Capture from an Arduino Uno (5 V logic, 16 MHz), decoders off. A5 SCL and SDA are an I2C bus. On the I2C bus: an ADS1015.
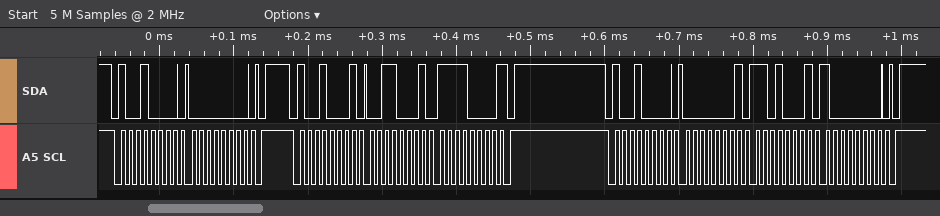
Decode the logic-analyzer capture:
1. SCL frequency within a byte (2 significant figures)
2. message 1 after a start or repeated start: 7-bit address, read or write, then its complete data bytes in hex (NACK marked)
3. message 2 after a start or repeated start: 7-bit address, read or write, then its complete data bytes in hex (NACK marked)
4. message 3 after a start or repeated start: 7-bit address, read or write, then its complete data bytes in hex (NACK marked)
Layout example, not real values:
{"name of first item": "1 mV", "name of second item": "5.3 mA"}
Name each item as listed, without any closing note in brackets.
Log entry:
{"SCL frequency within a byte": "100 kHz", "message 1 after a start or repeated start: 7-bit address, read or write, then its complete data bytes in hex": "0x48 write: 00", "message 2 after a start or repeated start: 7-bit address, read or write, then its complete data bytes in hex": "0x48 read: 31 F0 NACK", "message 3 after a start or repeated start: 7-bit address, read or write, then its complete data bytes in hex": "0x48 write: 01 D1 80"}
